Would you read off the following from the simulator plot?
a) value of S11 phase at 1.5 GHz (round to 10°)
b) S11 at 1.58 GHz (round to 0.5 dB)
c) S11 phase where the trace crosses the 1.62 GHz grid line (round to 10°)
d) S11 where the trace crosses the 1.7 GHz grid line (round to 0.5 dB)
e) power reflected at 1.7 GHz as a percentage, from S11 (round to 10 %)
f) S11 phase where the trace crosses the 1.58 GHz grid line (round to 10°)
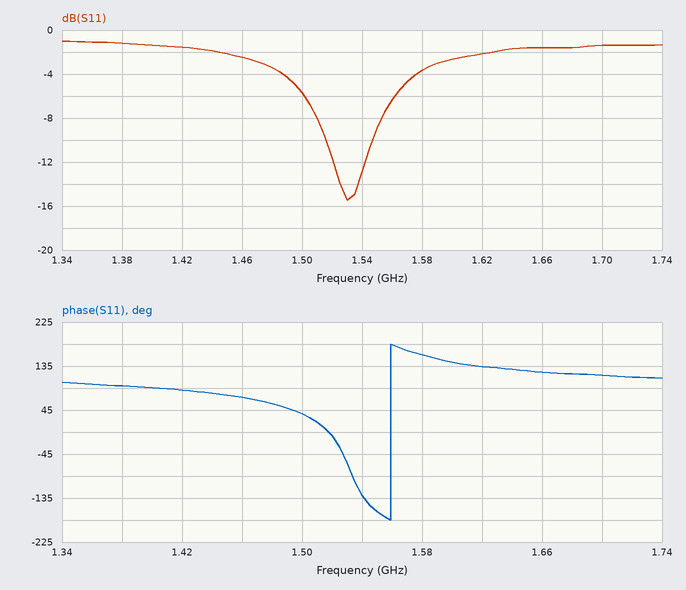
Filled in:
40°
-3.5 dB
130°
-1.5 dB
70 %
160°
